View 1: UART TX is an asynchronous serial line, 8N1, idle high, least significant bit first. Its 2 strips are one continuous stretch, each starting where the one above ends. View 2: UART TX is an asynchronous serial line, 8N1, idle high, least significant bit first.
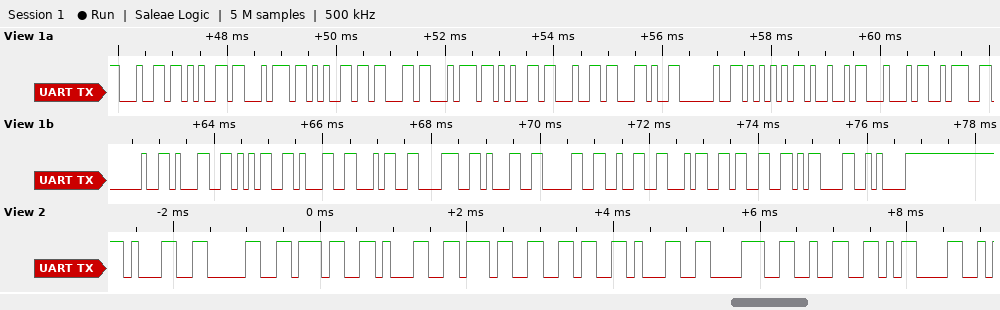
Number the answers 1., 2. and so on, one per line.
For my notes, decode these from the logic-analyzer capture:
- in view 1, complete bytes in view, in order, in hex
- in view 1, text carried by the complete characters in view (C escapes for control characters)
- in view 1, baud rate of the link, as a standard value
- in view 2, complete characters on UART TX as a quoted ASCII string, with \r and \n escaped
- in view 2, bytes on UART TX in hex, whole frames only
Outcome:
1. 64 65 74 65 63 74 65 64 2C 20 55 49 44 3A 20 31 35 31 34 38 31 30 32 34 33 0D 0A
2. "detected, UID: 1514810243\r\n"
3. 9600 baud
4. "107176182\r"
5. 31 30 37 31 37 36 31 38 32 0D
